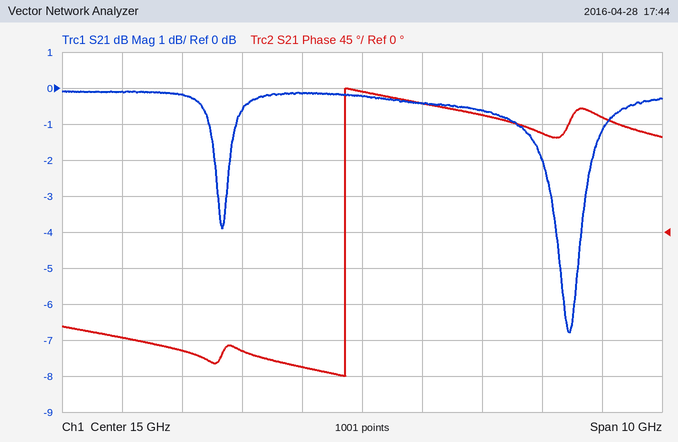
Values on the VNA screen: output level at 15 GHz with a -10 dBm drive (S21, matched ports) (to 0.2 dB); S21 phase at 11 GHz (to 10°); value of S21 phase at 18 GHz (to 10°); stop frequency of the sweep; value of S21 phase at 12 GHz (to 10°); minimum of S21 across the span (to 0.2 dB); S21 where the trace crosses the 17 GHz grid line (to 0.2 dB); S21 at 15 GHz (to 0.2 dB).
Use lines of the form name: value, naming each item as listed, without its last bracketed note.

output level at 15 GHz with a -10 dBm drive (S21, matched ports): -10.2 dBm
S21 phase at 11 GHz: -130°
value of S21 phase at 18 GHz: 120°
stop frequency of the sweep: 20 GHz
value of S21 phase at 12 GHz: -150°
minimum of S21 across the span: -6.8 dB
S21 where the trace crosses the 17 GHz grid line: -0.6 dB
S21 at 15 GHz: -0.2 dB
